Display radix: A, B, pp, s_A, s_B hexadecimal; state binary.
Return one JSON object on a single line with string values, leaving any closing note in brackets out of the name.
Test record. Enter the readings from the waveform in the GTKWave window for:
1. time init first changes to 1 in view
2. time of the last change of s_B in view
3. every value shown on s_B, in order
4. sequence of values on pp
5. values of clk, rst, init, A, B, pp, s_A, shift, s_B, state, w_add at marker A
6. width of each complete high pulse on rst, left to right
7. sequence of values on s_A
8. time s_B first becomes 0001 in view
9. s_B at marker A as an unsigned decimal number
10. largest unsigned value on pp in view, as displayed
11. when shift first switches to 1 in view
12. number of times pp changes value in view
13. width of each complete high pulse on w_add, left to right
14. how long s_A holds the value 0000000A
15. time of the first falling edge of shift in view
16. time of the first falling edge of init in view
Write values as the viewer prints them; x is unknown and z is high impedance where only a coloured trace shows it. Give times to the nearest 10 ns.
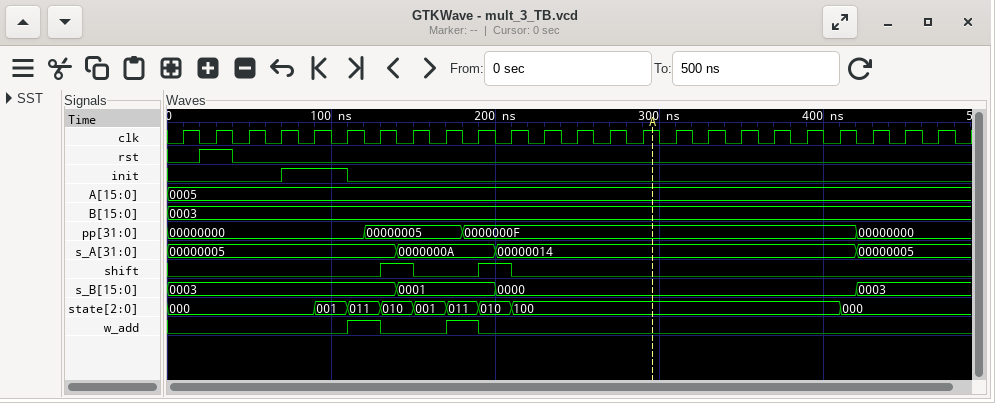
{"time init first changes to 1 in view": "70 ns", "time of the last change of s_B in view": "420 ns", "every value shown on s_B, in order": "0003, 0001, 0000, 0003", "sequence of values on pp": "00000000, 00000005, 0000000F, 00000000", "values of clk, rst, init, A, B, pp, s_A, shift, s_B, state, w_add at marker A": "clk=1, rst=0, init=0, A=0005, B=0003, pp=0000000F, s_A=00000014, shift=0, s_B=0000, state=100, w_add=0", "width of each complete high pulse on rst, left to right": "20 ns", "sequence of values on s_A": "00000005, 0000000A, 00000014, 00000005", "time s_B first becomes 0001 in view": "140 ns", "s_B at marker A as an unsigned decimal number": "0", "largest unsigned value on pp in view, as displayed": "0000000F", "when shift first switches to 1 in view": "130 ns", "number of times pp changes value in view": "3", "width of each complete high pulse on w_add, left to right": "20 ns, 20 ns", "how long s_A holds the value 0000000A": "60 ns", "time of the first falling edge of shift in view": "150 ns", "time of the first falling edge of init in view": "110 ns"}
